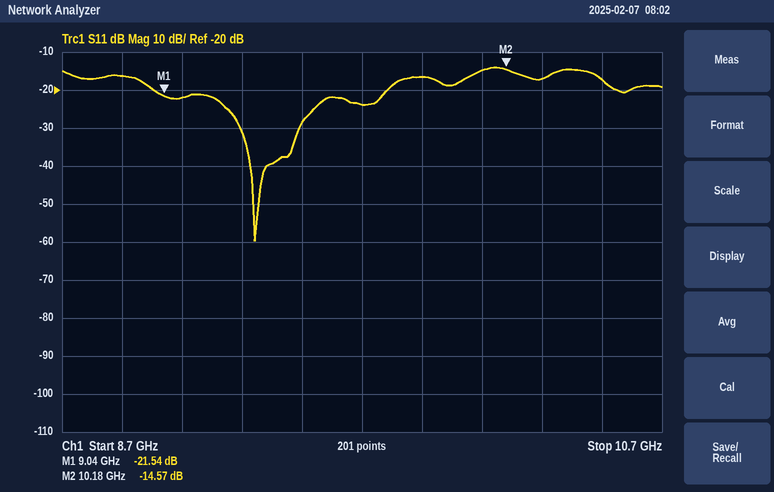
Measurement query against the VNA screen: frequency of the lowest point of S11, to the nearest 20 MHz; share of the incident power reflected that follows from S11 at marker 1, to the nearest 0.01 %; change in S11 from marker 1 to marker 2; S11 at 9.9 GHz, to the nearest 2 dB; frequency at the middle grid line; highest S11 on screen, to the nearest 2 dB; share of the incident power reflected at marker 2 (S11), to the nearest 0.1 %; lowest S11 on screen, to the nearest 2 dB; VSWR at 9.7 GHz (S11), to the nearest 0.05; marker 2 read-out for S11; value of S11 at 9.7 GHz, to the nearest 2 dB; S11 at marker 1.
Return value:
9.34 GHz
0.70 %
6.97 dB
-16 dB
9.7 GHz
-14 dB
3.5 %
-60 dB
1.15
-14.57 dB
-24 dB
-21.54 dB
